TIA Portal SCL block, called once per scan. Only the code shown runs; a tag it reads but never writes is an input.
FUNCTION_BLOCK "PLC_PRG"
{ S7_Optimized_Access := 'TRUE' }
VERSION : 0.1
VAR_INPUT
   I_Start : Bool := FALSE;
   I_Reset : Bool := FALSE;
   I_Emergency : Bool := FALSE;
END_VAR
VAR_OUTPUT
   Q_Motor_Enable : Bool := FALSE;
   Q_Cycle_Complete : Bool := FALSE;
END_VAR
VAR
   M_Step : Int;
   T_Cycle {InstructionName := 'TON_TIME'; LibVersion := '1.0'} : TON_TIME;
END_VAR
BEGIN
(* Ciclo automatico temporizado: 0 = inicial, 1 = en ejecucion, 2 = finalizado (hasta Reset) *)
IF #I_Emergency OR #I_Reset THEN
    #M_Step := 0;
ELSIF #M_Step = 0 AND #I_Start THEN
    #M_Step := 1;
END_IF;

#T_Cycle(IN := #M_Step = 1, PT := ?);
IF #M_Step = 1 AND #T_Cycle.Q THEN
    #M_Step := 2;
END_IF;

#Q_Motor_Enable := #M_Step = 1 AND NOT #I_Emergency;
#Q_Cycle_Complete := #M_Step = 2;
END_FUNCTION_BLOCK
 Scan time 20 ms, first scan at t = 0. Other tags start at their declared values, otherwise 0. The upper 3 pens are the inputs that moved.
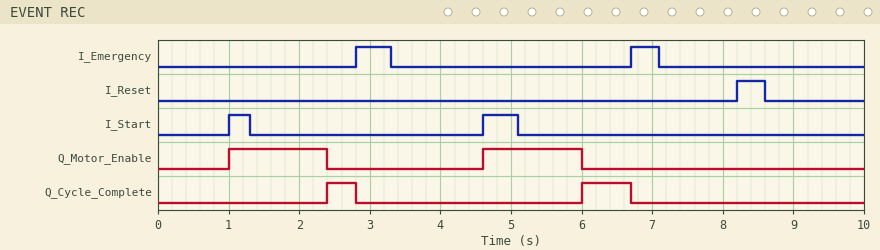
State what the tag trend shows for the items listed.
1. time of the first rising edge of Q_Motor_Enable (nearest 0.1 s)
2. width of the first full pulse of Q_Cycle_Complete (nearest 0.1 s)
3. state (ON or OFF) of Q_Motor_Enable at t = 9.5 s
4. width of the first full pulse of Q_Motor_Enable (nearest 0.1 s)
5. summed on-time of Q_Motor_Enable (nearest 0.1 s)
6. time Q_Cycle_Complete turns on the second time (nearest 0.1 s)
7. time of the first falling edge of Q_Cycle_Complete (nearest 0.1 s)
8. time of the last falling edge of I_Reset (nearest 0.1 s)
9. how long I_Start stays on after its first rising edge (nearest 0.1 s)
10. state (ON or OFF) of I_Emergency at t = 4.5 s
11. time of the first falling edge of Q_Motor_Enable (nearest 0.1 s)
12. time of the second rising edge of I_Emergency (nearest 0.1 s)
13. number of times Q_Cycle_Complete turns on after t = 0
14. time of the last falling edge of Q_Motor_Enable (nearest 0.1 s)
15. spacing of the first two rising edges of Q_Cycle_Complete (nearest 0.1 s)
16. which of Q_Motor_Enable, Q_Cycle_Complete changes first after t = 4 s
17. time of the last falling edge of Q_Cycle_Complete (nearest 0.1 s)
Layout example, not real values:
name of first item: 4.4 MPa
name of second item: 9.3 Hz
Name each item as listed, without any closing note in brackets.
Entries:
time of the first rising edge of Q_Motor_Enable: 1.0 s
width of the first full pulse of Q_Cycle_Complete: 0.4 s
state (ON or OFF) of Q_Motor_Enable at t = 9.5 s: OFF
width of the first full pulse of Q_Motor_Enable: 1.4 s
summed on-time of Q_Motor_Enable: 2.8 s
time Q_Cycle_Complete turns on the second time: 6.0 s
time of the first falling edge of Q_Cycle_Complete: 2.8 s
time of the last falling edge of I_Reset: 8.6 s
how long I_Start stays on after its first rising edge: 0.3 s
state (ON or OFF) of I_Emergency at t = 4.5 s: OFF
time of the first falling edge of Q_Motor_Enable: 2.4 s
time of the second rising edge of I_Emergency: 6.7 s
number of times Q_Cycle_Complete turns on after t = 0: 2
time of the last falling edge of Q_Motor_Enable: 6.0 s
spacing of the first two rising edges of Q_Cycle_Complete: 3.6 s
which of Q_Motor_Enable, Q_Cycle_Complete changes first after t = 4 s: Q_Motor_Enable
time of the last falling edge of Q_Cycle_Complete: 6.7 s
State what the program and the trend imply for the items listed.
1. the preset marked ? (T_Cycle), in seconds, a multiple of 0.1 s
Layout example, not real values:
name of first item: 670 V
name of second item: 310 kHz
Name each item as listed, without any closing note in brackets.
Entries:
the preset marked ? (T_Cycle), in seconds, a multiple of 0.1 s: 1.4 s
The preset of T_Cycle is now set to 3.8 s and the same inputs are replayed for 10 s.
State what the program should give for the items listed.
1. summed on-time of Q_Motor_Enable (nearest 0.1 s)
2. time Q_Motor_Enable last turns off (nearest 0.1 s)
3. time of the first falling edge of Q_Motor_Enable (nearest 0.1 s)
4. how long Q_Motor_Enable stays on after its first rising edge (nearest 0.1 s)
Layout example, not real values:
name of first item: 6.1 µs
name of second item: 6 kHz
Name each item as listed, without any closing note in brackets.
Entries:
summed on-time of Q_Motor_Enable: 3.9 s
time Q_Motor_Enable last turns off: 6.7 s
time of the first falling edge of Q_Motor_Enable: 2.8 s
how long Q_Motor_Enable stays on after its first rising edge: 1.8 s
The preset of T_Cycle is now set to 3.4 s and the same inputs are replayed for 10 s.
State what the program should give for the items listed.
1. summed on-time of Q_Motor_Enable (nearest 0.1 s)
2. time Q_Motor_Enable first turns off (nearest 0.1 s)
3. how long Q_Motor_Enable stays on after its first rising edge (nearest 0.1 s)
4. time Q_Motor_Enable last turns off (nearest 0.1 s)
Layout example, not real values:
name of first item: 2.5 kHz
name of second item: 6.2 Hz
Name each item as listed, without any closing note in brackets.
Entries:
summed on-time of Q_Motor_Enable: 3.9 s
time Q_Motor_Enable first turns off: 2.8 s
how long Q_Motor_Enable stays on after its first rising edge: 1.8 s
time Q_Motor_Enable last turns off: 6.7 s
